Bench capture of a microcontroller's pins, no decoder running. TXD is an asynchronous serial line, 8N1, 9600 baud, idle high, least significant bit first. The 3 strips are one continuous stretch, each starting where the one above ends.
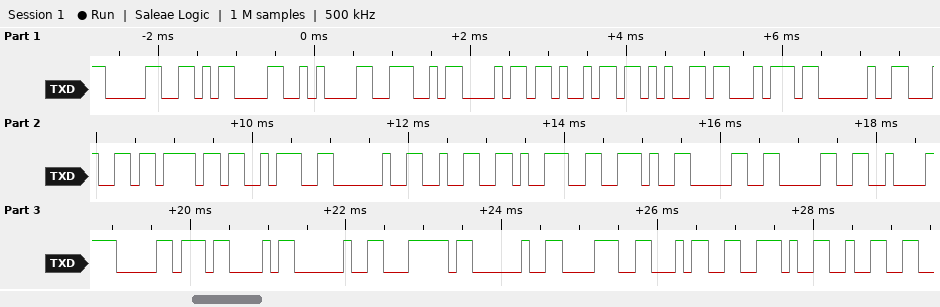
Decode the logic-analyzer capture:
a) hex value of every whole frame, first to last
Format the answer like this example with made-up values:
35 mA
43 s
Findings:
30 0D 0A 4E 68 69 65 74 20 64 6F 3A 20 32 39 2E 30 30 C2 B0 43 20 7C 20 38 34 2E 32
